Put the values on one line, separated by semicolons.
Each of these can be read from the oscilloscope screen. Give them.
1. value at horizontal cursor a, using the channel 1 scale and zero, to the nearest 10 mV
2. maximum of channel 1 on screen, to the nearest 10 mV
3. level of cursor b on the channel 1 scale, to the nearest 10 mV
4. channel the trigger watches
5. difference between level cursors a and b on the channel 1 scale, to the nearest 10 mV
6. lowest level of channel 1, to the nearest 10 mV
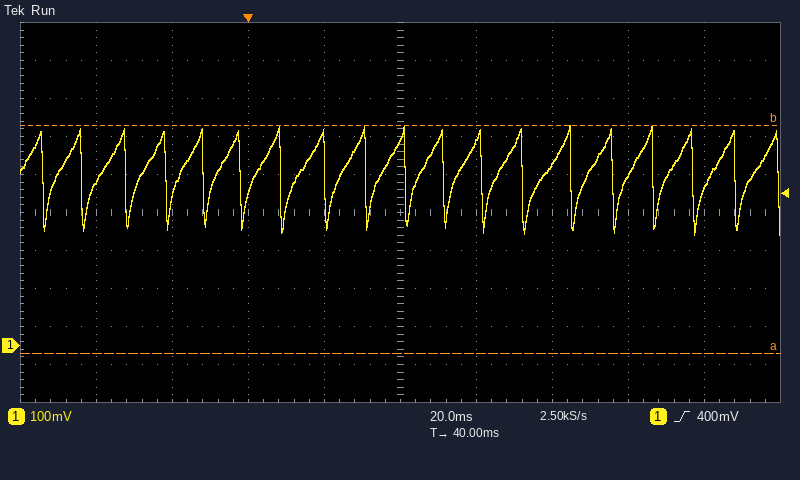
-20 mV; 580 mV; 580 mV; channel 1; 600 mV; 290 mV
